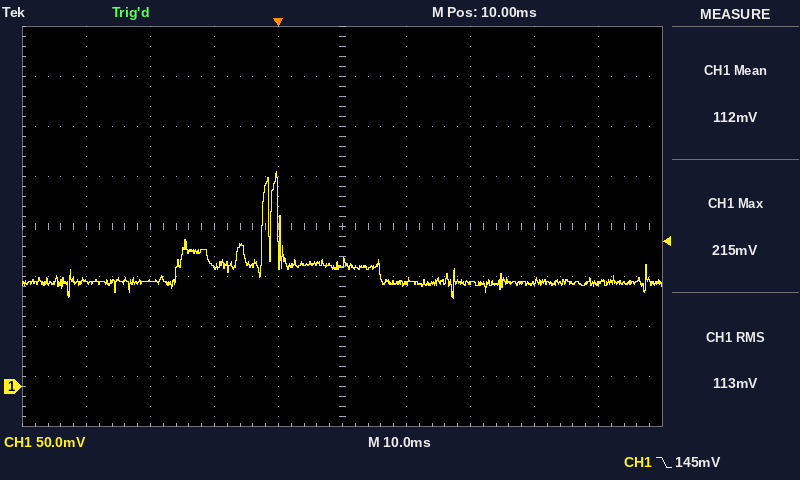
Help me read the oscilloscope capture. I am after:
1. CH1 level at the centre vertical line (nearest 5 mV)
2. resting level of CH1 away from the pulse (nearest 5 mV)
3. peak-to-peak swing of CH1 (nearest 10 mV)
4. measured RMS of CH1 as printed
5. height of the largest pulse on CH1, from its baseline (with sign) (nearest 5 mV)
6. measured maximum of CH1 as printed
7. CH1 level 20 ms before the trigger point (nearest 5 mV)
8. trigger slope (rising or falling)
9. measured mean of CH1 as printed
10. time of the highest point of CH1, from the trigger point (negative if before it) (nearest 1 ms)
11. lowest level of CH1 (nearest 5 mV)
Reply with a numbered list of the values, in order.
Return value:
1. 125 mV
2. 105 mV
3. 130 mV
4. 113 mV
5. +110 mV
6. 215 mV
7. 105 mV
8. falling
9. 112 mV
10. 0 ms
11. 90 mV
